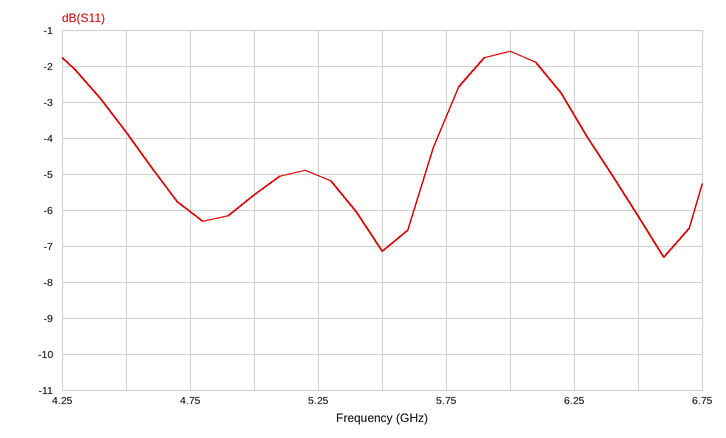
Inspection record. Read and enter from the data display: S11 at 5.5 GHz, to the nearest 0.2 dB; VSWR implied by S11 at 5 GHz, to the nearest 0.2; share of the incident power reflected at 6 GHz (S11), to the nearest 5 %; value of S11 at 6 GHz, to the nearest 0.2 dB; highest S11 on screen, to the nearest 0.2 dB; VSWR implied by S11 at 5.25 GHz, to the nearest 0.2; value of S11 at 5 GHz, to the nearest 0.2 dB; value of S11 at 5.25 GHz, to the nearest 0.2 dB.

-7.2 dB
3.2
70 %
-1.6 dB
-1.6 dB
3.6
-5.6 dB
-5.0 dB
